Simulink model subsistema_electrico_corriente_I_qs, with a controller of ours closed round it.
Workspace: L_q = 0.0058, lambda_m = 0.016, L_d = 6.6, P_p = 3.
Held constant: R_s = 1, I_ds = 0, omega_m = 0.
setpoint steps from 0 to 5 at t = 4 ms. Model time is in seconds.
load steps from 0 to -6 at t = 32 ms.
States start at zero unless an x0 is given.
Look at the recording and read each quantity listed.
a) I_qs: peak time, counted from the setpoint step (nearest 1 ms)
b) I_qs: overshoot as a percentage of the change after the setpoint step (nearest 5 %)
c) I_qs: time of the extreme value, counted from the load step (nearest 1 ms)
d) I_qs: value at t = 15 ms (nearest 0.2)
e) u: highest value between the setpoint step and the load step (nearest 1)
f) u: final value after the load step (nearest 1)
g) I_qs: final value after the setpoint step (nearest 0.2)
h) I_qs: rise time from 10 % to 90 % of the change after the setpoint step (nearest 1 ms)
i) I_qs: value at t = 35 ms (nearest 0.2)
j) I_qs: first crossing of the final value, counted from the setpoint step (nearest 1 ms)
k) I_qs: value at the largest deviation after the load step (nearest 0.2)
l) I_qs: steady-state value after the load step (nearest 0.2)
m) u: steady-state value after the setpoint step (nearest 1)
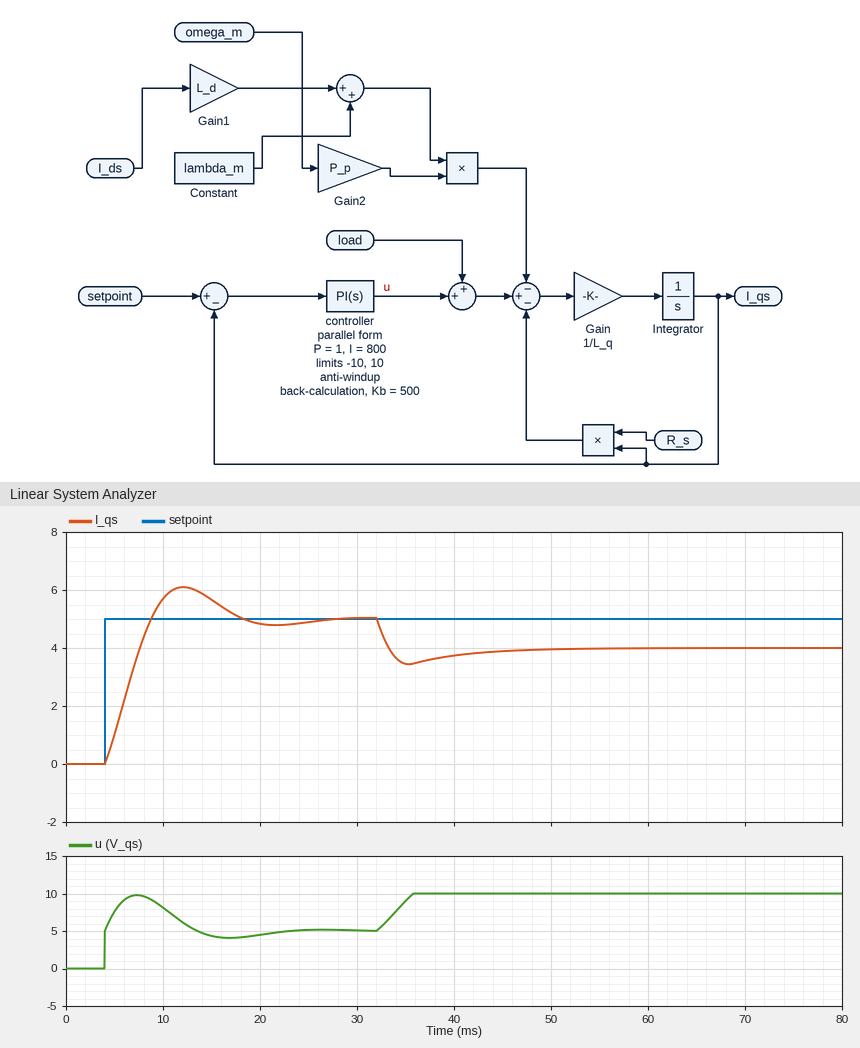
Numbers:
8 ms
20 %
3 ms
5.6
10
10
5.0
4 ms
3.4
5 ms
3.4
4.0
5
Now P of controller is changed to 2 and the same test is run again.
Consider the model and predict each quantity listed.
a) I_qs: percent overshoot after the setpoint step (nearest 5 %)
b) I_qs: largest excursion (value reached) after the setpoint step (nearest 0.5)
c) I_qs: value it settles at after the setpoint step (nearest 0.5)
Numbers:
10 %
5.5
5.0
